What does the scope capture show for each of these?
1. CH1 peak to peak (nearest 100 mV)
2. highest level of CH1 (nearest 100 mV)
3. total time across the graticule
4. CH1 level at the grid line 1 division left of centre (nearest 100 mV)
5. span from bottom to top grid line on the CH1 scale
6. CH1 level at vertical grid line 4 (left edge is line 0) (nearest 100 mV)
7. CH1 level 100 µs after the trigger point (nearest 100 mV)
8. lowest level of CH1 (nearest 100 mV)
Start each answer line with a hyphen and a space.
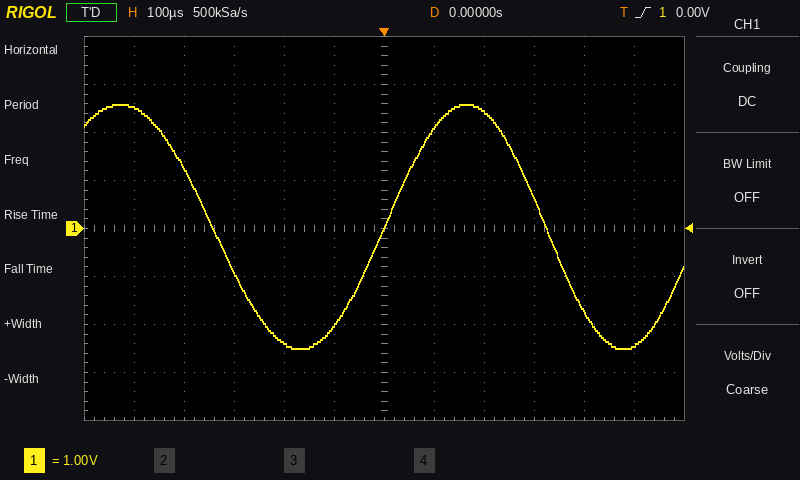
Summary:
- 5.1 V
- 2.6 V
- 1.2 ms
- -2.0 V
- 8 V
- -2.4 V
- 2.1 V
- -2.5 V
